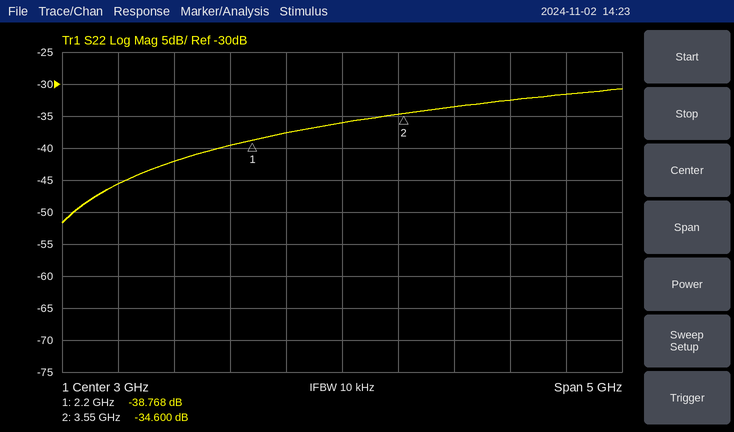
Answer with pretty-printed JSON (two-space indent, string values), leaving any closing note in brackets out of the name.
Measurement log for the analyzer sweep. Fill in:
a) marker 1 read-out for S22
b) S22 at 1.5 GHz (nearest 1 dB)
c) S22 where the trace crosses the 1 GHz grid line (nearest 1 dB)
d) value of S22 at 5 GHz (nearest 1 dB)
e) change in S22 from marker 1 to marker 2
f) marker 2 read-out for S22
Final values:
{
  "marker 1 read-out for S22": "-38.768 dB",
  "S22 at 1.5 GHz": "-42 dB",
  "S22 where the trace crosses the 1 GHz grid line": "-46 dB",
  "value of S22 at 5 GHz": "-32 dB",
  "change in S22 from marker 1 to marker 2": "4.168 dB",
  "marker 2 read-out for S22": "-34.600 dB"
}
